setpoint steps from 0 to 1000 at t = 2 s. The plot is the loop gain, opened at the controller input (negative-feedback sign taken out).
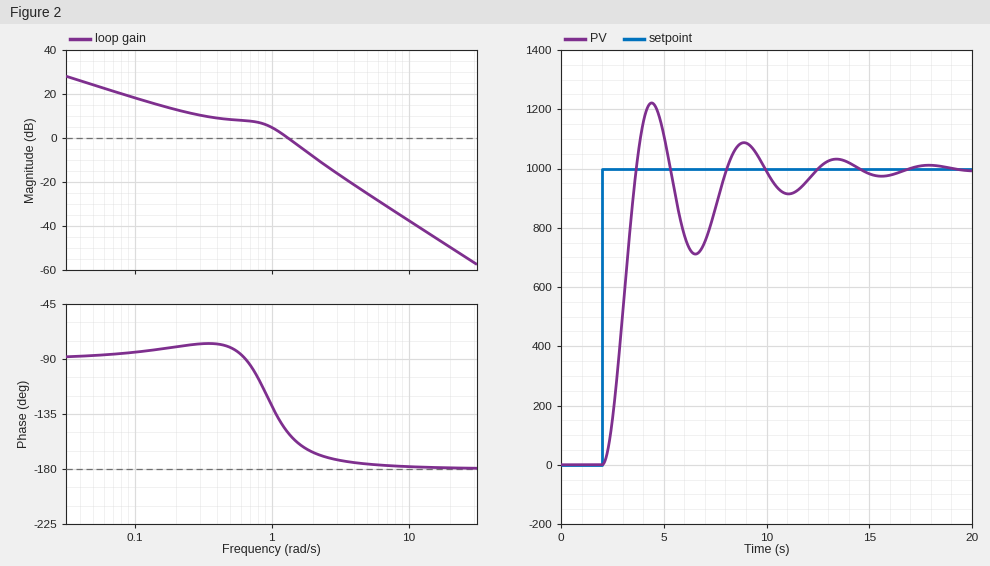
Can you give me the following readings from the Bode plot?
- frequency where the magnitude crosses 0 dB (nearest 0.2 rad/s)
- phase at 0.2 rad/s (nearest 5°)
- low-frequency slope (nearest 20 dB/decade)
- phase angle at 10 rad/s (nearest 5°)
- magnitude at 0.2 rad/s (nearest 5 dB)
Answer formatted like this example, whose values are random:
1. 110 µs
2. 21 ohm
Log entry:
1. 1.4 rad/s
2. -80°
3. -20 dB/decade
4. -180°
5. 15 dB
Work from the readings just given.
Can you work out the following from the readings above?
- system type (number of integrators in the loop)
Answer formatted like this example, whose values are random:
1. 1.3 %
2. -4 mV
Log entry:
1. 1
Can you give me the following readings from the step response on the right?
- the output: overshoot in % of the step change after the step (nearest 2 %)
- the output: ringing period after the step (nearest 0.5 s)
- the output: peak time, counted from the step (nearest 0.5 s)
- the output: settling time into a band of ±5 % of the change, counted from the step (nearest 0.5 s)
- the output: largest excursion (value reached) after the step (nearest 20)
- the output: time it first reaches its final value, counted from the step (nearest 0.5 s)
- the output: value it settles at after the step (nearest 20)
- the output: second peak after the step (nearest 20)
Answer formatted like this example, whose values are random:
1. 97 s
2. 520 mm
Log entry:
1. 22 %
2. 4.5 s
3. 2.5 s
4. 10.0 s
5. 1220
6. 1.5 s
7. 1000
8. 1080
